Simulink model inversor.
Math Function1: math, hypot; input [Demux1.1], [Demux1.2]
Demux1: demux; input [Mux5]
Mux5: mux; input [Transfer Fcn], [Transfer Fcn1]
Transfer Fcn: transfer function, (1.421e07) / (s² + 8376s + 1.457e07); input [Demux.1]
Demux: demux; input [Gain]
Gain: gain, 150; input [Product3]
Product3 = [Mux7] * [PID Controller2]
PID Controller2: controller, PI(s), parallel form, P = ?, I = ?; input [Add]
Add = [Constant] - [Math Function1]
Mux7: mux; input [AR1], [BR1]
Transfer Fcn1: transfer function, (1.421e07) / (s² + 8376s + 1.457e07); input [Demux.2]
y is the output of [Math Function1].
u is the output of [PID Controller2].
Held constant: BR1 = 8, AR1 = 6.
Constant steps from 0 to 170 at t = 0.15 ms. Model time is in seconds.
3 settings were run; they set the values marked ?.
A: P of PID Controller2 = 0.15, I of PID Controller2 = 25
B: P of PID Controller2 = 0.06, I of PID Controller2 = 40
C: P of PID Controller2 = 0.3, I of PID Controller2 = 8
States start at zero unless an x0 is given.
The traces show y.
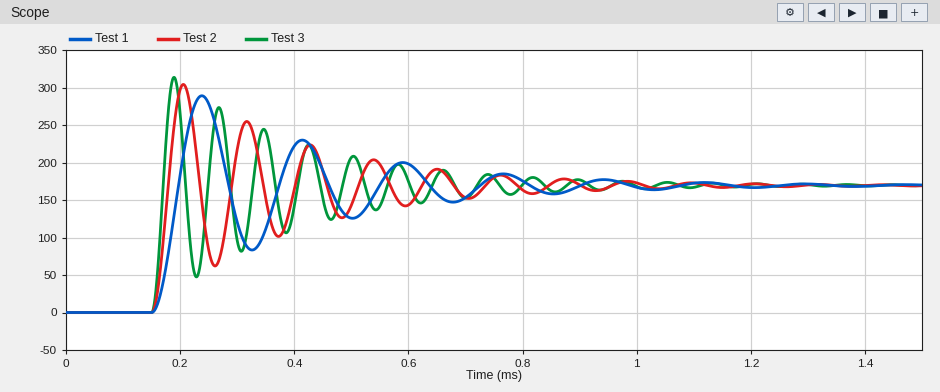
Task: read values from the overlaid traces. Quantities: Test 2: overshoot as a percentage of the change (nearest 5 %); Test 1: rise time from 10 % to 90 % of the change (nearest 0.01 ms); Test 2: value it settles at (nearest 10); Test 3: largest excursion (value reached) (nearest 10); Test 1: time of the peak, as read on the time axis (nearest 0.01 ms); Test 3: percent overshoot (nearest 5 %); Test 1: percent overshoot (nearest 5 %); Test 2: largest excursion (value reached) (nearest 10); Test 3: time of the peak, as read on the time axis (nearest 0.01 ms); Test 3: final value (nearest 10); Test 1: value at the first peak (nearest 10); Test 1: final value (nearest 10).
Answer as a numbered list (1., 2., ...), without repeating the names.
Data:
1. 80 %
2. 0.03 ms
3. 170
4. 310
5. 0.24 ms
6. 85 %
7. 70 %
8. 300
9. 0.19 ms
10. 170
11. 290
12. 170
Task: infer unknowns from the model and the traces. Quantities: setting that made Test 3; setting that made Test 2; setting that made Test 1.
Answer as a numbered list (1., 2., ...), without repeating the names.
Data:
1. C
2. A
3. B
